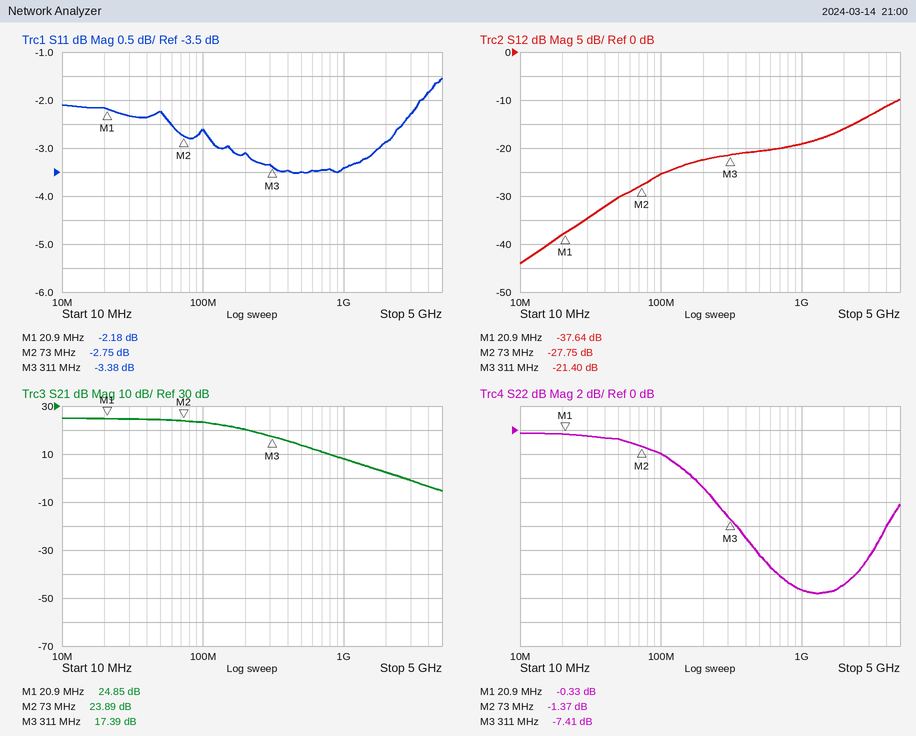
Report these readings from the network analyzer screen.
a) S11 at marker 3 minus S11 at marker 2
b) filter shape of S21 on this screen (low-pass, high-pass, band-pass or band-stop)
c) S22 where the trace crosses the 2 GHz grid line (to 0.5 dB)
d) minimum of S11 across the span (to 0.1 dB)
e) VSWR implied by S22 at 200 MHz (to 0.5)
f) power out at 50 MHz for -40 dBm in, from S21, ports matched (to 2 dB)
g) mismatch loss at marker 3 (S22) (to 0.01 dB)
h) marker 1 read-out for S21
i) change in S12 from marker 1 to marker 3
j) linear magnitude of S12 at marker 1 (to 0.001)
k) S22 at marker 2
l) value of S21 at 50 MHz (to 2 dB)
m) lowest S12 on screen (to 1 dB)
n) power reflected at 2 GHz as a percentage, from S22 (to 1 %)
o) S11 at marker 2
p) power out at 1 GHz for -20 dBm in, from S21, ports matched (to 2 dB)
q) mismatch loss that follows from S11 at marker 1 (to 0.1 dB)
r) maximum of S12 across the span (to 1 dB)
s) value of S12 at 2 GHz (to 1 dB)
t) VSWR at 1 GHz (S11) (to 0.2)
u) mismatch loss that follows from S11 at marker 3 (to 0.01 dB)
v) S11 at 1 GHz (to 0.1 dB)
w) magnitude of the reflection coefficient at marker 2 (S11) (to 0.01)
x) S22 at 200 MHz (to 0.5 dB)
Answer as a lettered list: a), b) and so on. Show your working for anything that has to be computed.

a) -3.38 − (-2.75) = -0.63 dB
b) low-pass
c) -13.0 dB
d) -3.5 dB
e) |Γ| = 10^(-5/20) = 0.5623; VSWR = (1 + 0.5623)/(1 − 0.5623) ≈ 3.57, so 3.5 to the nearest 0.5
f) -40 dBm + (24 dB) = -16 dBm
g) −10 log10(1 − 10^(-7.41/10)) ≈ 0.87 dB
h) 24.85 dB
i) -21.4 − (-37.64) = 16.24 dB
j) 10^(-37.64/20) ≈ 0.013
k) -1.37 dB
l) 24 dB
m) -44 dB
n) 10^(-13/10) ≈ 5 %
o) -2.75 dB
p) -20 dBm + (8 dB) = -12 dBm
q) −10 log10(1 − 10^(-2.18/10)) ≈ 4.0 dB
r) -10 dB
s) -16 dB
t) |Γ| = 10^(-3.4/20) = 0.6761; VSWR = (1 + 0.6761)/(1 − 0.6761) ≈ 5.2
u) −10 log10(1 − 10^(-3.38/10)) ≈ 2.67 dB
v) -3.4 dB
w) 10^(-2.75/20) ≈ 0.73
x) -5.0 dB
